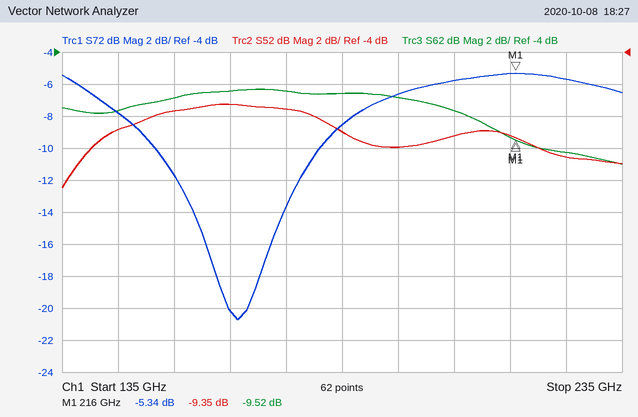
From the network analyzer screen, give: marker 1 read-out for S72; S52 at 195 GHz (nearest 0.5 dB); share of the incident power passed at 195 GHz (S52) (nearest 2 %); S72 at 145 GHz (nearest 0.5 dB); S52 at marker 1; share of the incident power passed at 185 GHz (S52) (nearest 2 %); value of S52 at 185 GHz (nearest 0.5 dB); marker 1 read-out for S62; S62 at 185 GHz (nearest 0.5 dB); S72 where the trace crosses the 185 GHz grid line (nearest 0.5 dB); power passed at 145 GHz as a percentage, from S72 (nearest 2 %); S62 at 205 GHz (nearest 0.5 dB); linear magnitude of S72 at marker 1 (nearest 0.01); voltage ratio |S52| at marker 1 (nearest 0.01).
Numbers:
-5.34 dB
-10.0 dB
10 %
-8.0 dB
-9.35 dB
12 %
-9.0 dB
-9.52 dB
-6.5 dB
-8.5 dB
16 %
-7.5 dB
0.54
0.34
